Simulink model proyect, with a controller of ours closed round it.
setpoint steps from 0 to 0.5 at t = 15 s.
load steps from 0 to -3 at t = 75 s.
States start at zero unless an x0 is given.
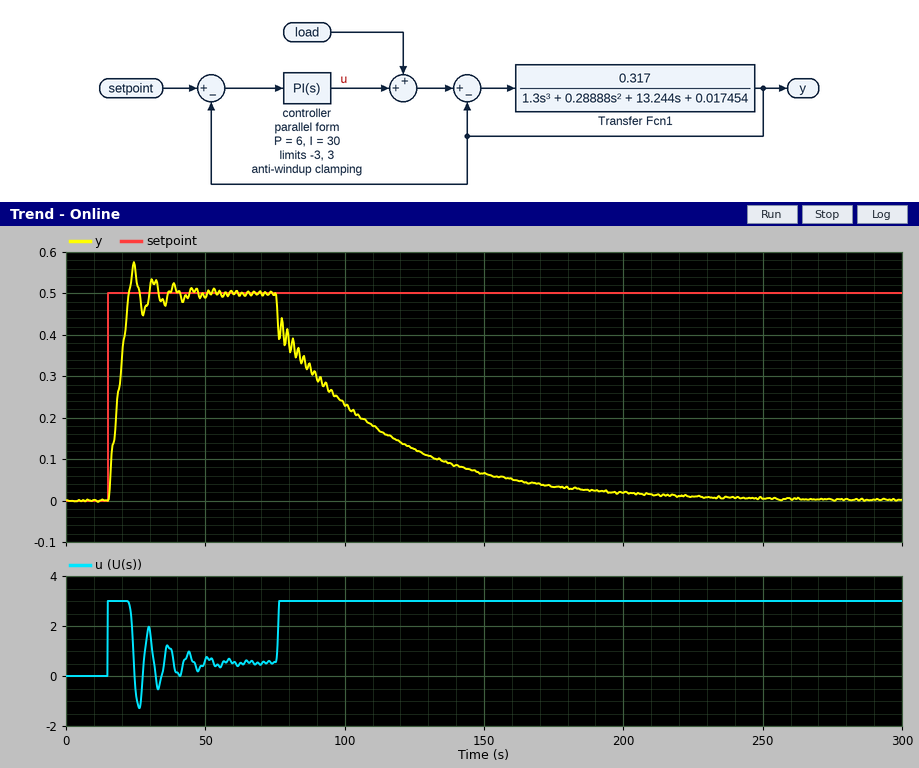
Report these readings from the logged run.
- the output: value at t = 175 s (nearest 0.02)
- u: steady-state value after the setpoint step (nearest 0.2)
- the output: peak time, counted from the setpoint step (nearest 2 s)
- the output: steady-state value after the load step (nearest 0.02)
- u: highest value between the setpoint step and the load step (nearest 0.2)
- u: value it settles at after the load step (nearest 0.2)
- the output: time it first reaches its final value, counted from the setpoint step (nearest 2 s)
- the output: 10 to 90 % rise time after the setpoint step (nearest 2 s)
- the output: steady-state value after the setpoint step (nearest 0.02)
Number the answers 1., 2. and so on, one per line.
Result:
1. 0.04
2. 0.6
3. 10 s
4. 0.00
5. 3.0
6. 3.0
7. 8 s
8. 6 s
9. 0.50
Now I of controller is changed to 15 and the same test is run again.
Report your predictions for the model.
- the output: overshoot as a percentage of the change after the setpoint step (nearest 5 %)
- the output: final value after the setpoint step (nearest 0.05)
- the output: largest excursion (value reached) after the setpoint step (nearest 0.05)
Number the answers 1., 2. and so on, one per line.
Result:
1. 15 %
2. 0.50
3. 0.60
